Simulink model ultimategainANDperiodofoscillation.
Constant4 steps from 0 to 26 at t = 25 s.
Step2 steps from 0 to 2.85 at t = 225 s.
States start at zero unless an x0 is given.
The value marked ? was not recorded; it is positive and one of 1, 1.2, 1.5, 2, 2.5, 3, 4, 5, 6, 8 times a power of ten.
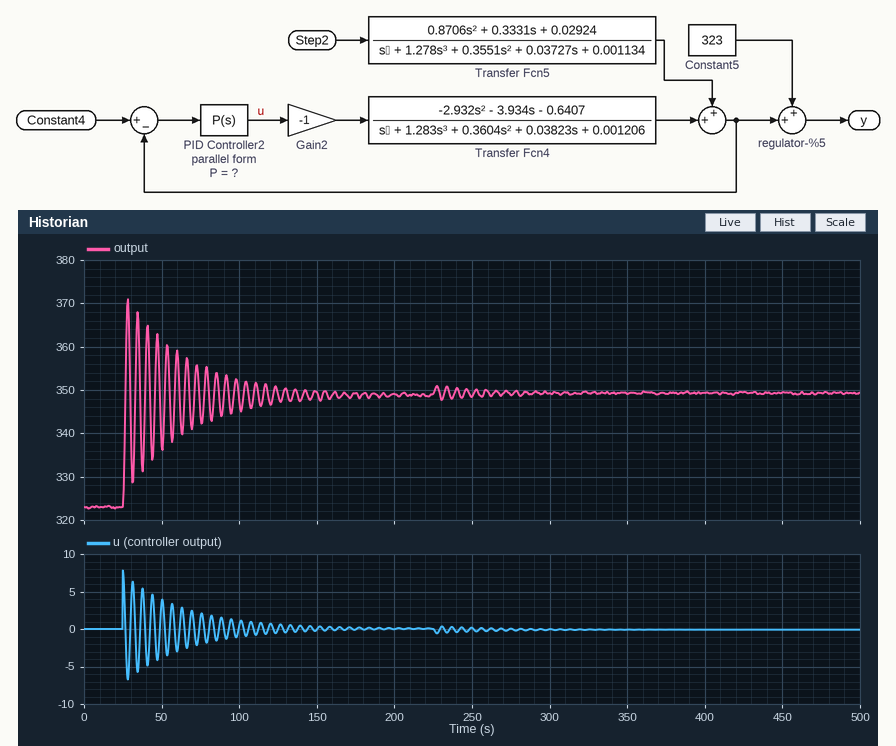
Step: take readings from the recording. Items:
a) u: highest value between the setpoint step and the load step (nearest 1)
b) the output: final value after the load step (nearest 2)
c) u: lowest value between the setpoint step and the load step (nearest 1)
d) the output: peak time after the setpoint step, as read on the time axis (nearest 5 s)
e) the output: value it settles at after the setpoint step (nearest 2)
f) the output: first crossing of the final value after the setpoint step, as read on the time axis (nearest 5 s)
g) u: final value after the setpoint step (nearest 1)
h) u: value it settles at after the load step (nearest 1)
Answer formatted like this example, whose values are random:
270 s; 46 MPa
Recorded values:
8; 350; -7; 30 s; 348; 25 s; 0; 0
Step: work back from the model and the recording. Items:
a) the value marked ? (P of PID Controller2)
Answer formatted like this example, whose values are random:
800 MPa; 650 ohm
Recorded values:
0.3
